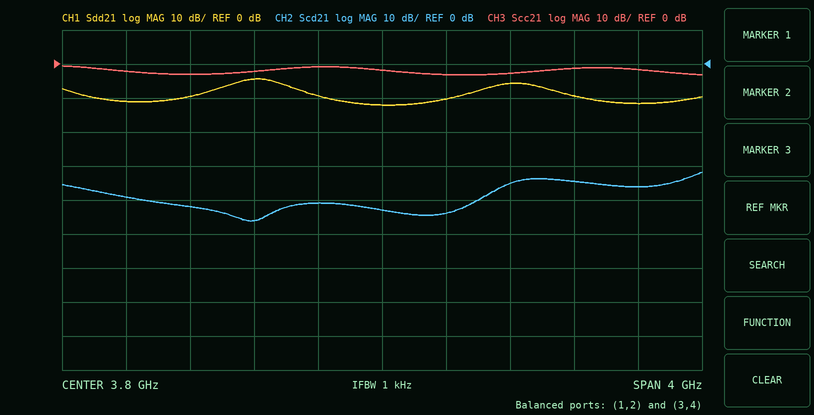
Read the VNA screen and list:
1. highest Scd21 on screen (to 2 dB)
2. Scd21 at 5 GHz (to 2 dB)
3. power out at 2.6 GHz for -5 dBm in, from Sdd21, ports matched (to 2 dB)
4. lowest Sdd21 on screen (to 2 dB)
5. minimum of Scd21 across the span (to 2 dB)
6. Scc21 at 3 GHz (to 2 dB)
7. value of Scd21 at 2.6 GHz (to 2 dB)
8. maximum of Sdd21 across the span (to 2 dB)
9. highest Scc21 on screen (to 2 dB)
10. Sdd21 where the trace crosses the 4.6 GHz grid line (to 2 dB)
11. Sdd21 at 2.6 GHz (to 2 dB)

-32 dB
-34 dB
-14 dBm
-12 dB
-46 dB
-2 dB
-42 dB
-4 dB
0 dB
-6 dB
-10 dB
